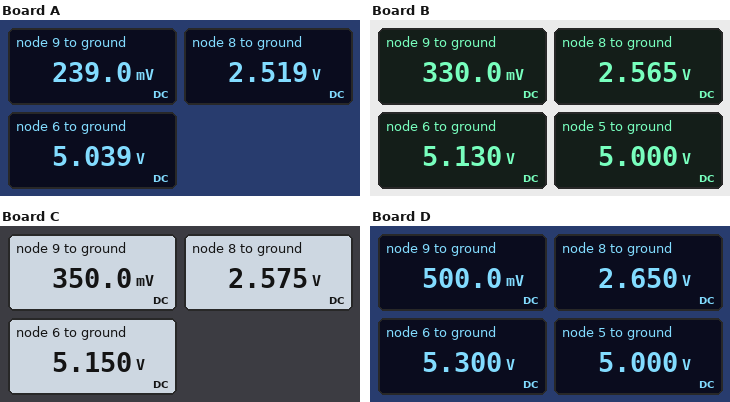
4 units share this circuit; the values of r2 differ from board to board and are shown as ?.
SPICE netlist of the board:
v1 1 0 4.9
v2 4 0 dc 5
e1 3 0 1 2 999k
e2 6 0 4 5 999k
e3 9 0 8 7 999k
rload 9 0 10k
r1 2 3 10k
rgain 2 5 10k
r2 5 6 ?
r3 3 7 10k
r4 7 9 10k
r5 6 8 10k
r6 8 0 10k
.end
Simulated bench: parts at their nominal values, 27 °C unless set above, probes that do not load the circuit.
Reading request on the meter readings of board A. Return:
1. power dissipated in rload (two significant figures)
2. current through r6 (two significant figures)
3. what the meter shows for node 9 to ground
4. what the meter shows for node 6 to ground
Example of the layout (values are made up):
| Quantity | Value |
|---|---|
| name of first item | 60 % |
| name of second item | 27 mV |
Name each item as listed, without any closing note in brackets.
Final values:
| Quantity | Value |
|---|---|
| power dissipated in rload | 5.7 µW |
| current through r6 | 250 µA |
| what the meter shows for node 9 to ground | 239.0 mV |
| what the meter shows for node 6 to ground | 5.039 V |
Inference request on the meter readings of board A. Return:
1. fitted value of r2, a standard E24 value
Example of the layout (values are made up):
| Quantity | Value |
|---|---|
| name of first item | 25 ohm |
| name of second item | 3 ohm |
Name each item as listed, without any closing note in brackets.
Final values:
| Quantity | Value |
|---|---|
| fitted value of r2, a standard E24 value | 3.9 kΩ |
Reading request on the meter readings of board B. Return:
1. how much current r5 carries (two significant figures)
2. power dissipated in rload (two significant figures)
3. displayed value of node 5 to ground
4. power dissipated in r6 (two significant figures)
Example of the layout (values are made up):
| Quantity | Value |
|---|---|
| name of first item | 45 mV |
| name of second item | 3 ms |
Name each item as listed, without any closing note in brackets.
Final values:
| Quantity | Value |
|---|---|
| how much current r5 carries | 260 µA |
| power dissipated in rload | 11 µW |
| displayed value of node 5 to ground | 5.000 V |
| power dissipated in r6 | 660 µW |
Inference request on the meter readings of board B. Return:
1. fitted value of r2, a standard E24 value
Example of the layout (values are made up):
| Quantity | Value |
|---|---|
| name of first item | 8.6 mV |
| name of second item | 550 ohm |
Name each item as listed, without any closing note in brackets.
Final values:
| Quantity | Value |
|---|---|
| fitted value of r2, a standard E24 value | 13 kΩ |
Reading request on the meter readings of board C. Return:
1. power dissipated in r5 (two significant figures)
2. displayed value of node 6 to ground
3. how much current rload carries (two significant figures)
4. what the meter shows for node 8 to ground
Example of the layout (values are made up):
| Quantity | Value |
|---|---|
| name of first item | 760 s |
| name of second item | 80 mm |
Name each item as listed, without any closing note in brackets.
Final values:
| Quantity | Value |
|---|---|
| power dissipated in r5 | 660 µW |
| displayed value of node 6 to ground | 5.150 V |
| how much current rload carries | 35 µA |
| what the meter shows for node 8 to ground | 2.575 V |
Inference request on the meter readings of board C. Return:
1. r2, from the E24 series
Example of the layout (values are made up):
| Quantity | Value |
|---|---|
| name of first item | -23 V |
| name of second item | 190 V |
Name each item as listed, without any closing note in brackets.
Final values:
| Quantity | Value |
|---|---|
| r2, from the E24 series | 15 kΩ |
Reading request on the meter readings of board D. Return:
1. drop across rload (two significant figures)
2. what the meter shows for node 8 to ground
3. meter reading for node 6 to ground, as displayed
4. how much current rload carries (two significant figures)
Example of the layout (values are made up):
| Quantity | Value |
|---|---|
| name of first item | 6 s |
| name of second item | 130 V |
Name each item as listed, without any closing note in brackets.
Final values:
| Quantity | Value |
|---|---|
| drop across rload | 500 mV |
| what the meter shows for node 8 to ground | 2.650 V |
| meter reading for node 6 to ground, as displayed | 5.300 V |
| how much current rload carries | 50 µA |
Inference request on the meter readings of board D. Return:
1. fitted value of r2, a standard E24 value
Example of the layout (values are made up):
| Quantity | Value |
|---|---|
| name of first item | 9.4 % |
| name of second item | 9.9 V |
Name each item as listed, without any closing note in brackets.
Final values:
| Quantity | Value |
|---|---|
| fitted value of r2, a standard E24 value | 30 kΩ |
